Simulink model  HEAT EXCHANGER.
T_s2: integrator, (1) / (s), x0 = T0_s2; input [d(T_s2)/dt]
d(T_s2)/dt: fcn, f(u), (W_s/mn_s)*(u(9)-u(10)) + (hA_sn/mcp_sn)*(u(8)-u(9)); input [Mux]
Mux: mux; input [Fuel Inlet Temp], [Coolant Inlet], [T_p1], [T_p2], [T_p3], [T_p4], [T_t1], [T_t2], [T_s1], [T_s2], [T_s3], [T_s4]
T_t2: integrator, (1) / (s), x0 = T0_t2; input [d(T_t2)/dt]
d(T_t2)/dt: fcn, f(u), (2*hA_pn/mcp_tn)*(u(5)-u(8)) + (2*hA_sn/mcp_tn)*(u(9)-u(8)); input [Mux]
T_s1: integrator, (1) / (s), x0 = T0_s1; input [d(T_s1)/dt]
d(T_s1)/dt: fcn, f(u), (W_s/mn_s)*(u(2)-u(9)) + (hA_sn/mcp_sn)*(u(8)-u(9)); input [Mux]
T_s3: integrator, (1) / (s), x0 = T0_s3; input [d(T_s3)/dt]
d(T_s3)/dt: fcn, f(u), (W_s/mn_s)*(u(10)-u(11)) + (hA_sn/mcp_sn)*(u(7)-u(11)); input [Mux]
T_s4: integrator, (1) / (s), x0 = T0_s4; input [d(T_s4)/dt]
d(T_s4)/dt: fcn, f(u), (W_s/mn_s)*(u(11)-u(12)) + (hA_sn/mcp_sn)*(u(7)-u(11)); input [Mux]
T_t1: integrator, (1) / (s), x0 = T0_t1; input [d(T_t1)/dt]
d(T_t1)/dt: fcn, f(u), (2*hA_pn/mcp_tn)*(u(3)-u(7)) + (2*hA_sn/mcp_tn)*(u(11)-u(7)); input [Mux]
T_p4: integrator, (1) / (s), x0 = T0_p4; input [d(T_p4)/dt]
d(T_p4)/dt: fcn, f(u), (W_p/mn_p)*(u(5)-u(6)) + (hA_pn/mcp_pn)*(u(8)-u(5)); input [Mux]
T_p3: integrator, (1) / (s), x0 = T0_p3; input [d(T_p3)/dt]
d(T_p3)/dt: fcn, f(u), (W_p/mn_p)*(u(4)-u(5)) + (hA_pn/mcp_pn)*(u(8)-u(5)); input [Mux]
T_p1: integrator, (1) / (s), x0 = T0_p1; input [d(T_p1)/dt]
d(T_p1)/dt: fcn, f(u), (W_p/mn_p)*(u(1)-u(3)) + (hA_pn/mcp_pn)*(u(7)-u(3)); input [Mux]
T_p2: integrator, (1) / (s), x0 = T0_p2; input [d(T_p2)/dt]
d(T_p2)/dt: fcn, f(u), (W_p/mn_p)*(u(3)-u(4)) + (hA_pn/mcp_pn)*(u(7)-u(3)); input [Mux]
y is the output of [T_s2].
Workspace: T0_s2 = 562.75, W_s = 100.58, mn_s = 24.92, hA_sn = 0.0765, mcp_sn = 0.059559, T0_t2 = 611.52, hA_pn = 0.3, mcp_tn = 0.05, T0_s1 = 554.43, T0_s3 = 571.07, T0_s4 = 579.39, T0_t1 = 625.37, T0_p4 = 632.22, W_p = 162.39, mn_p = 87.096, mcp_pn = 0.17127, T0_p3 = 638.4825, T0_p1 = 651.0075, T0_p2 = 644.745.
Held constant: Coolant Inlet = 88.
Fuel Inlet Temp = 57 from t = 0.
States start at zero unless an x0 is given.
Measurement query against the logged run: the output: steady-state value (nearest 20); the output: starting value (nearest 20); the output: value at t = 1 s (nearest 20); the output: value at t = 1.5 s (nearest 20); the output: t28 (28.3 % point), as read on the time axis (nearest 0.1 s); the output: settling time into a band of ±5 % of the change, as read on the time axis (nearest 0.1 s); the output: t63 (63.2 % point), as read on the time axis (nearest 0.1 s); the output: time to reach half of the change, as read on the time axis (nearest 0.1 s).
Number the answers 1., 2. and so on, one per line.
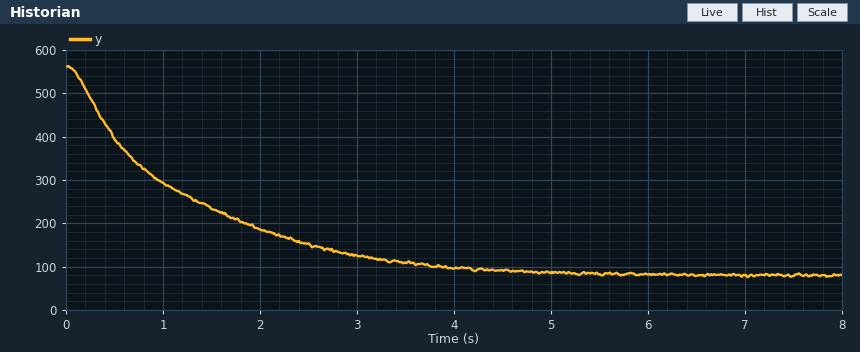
1. 80
2. 560
3. 300
4. 240
5. 0.4 s
6. 3.7 s
7. 1.3 s
8. 0.8 s
